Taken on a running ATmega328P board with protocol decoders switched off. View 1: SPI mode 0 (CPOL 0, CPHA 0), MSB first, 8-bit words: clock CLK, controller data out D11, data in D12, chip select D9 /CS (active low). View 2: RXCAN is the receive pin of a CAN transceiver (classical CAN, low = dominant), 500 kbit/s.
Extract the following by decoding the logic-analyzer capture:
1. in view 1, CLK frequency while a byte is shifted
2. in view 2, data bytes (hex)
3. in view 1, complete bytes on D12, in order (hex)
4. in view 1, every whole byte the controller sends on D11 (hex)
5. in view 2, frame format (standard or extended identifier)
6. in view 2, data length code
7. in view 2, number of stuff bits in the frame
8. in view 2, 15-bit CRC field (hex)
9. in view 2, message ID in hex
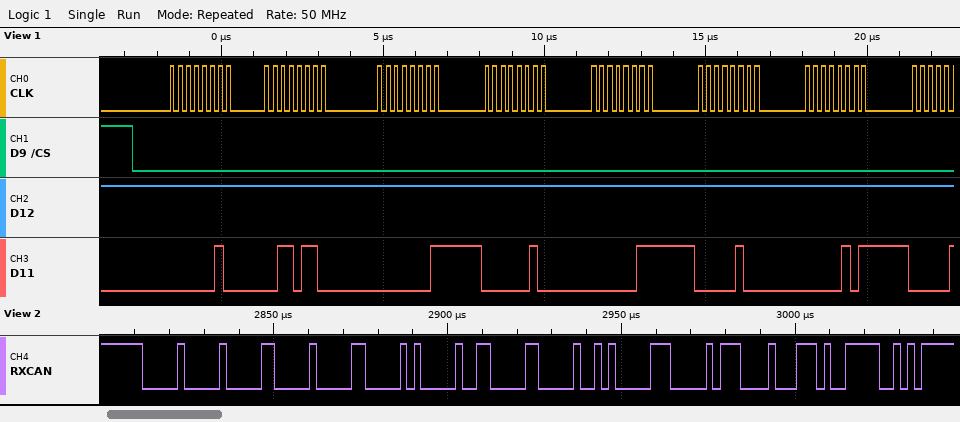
4 MHz
01 02 03 04 05 06 07 08
0xFF 0xFF 0xFF 0xFF 0xFF 0xFF 0xFF
0x02 0x36 0x01 0x02 0x03 0x04 0x05
standard
8
12
0x74FA
0x000
